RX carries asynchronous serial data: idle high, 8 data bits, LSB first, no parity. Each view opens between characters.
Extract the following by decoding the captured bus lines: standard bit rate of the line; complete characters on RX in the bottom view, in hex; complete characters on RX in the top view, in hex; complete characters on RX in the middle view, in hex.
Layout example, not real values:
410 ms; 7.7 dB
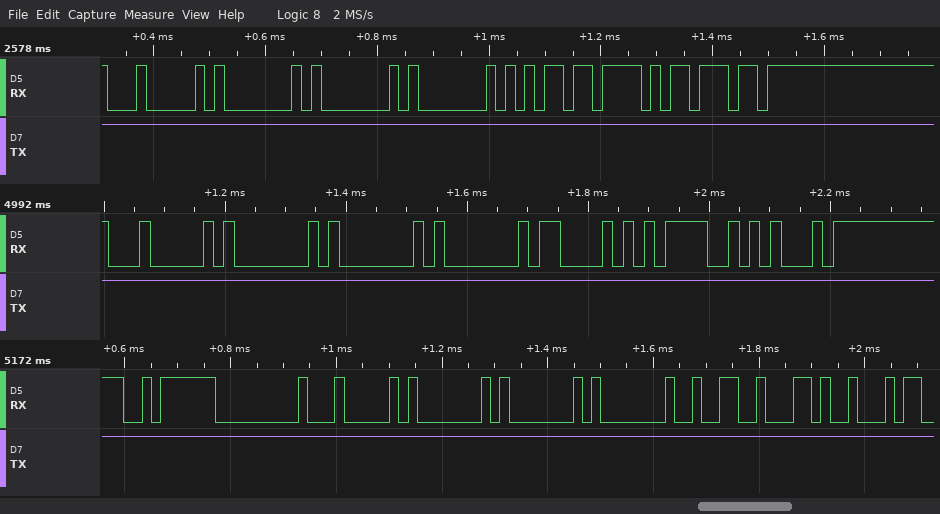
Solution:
57600 baud; FA, 00, 04, 01, 01, 01, 32, 2C; 04, 01, 01, 01, B5, AF, B7; 04, 01, 01, 01, 43, 3D, 45
